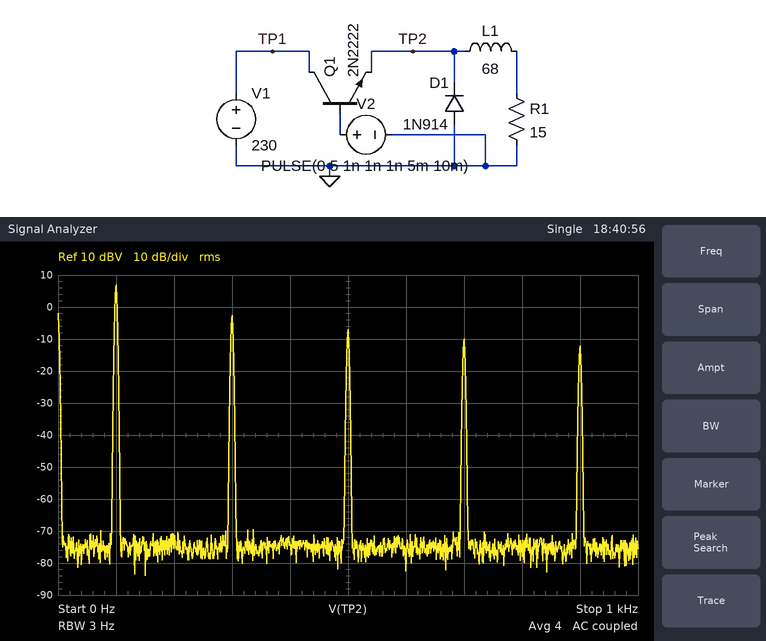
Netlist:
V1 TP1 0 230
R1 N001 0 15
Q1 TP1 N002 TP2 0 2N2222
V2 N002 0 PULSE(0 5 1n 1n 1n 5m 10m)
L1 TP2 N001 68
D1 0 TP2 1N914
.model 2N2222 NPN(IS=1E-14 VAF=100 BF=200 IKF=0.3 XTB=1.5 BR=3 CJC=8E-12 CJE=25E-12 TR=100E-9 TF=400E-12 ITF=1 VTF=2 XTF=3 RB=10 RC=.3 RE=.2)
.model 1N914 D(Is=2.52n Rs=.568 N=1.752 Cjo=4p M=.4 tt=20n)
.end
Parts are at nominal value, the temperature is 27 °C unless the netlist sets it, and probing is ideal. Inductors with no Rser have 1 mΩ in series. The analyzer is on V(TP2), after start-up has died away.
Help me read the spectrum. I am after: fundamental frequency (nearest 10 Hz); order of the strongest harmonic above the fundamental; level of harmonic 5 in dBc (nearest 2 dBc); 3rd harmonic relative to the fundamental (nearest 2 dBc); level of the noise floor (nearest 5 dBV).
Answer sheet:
100 Hz
3
-14 dBc
-10 dBc
-75 dBV
